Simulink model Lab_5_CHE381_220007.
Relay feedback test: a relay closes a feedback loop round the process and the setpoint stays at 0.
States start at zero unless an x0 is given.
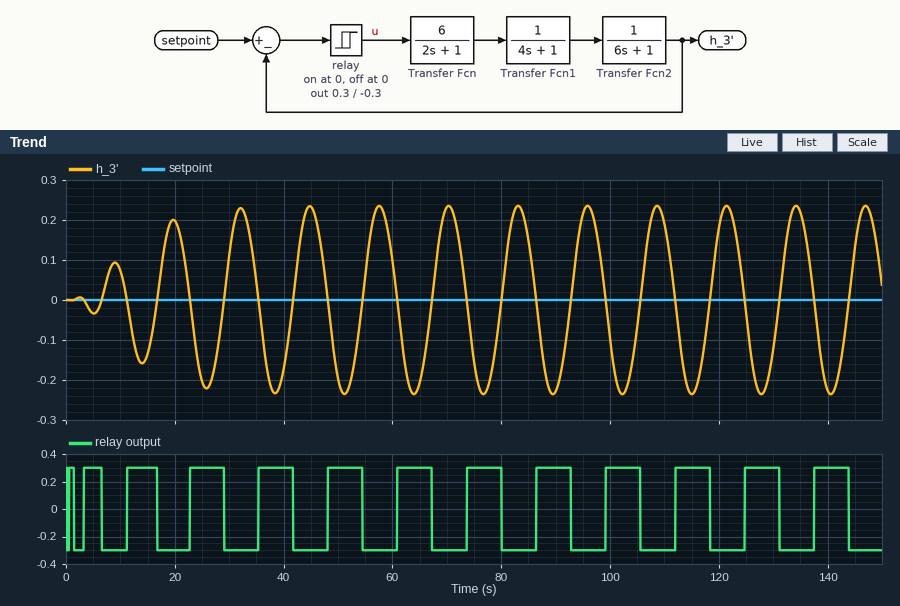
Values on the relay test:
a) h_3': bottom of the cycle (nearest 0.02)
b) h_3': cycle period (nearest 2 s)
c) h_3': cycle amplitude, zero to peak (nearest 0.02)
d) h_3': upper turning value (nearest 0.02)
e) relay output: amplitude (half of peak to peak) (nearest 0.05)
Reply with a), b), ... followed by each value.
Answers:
a) -0.24
b) 12 s
c) 0.24
d) 0.24
e) 0.30
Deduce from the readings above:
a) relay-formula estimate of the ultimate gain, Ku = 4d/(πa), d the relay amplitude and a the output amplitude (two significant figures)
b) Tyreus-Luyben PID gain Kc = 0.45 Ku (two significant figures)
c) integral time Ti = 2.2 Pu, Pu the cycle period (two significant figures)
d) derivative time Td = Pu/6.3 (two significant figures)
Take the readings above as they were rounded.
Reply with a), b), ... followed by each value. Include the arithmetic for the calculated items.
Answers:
a) 4 × 0.3 / (π × 0.24) = 1.6
b) 0.45 × 1.6 = 0.72
c) 2.2 × 12 = 26 s
d) 12 / 6.3 = 1.9 s
